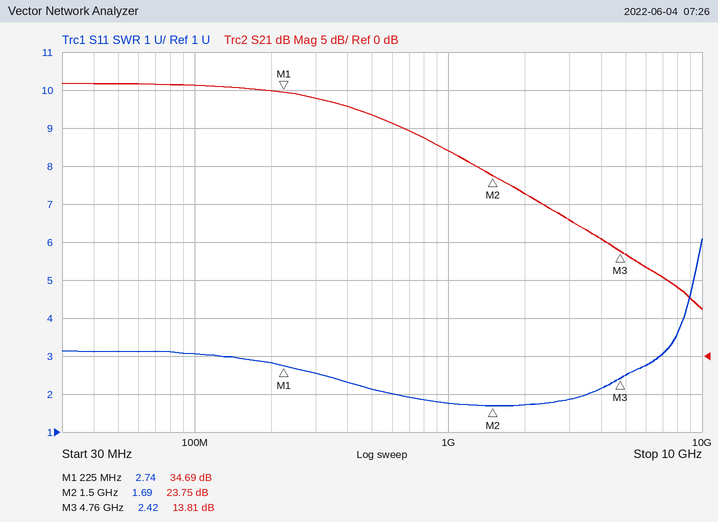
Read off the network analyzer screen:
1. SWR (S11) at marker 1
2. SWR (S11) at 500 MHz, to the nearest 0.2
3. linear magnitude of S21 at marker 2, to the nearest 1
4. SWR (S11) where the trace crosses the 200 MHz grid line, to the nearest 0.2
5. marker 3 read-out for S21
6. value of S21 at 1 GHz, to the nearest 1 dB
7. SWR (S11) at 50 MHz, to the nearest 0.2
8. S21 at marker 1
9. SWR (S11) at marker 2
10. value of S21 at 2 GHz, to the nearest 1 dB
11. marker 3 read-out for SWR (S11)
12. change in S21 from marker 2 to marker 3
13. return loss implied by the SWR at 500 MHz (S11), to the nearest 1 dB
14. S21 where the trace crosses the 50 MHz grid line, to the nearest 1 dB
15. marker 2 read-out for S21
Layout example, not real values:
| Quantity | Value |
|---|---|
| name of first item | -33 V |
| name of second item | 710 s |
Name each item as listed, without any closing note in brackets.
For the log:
| Quantity | Value |
|---|---|
| SWR (S11) at marker 1 | 2.74 |
| SWR (S11) at 500 MHz, to the nearest 0.2 | 2.2 |
| linear magnitude of S21 at marker 2, to the nearest 1 | 15 |
| SWR (S11) where the trace crosses the 200 MHz grid line, to the nearest 0.2 | 2.8 |
| marker 3 read-out for S21 | 13.81 dB |
| value of S21 at 1 GHz, to the nearest 1 dB | 27 dB |
| SWR (S11) at 50 MHz, to the nearest 0.2 | 3.2 |
| S21 at marker 1 | 34.69 dB |
| SWR (S11) at marker 2 | 1.69 |
| value of S21 at 2 GHz, to the nearest 1 dB | 21 dB |
| marker 3 read-out for SWR | 2.42 |
| change in S21 from marker 2 to marker 3 | -9.94 dB |
| return loss implied by the SWR at 500 MHz (S11), to the nearest 1 dB | 9 dB |
| S21 where the trace crosses the 50 MHz grid line, to the nearest 1 dB | 36 dB |
| marker 2 read-out for S21 | 23.75 dB |
